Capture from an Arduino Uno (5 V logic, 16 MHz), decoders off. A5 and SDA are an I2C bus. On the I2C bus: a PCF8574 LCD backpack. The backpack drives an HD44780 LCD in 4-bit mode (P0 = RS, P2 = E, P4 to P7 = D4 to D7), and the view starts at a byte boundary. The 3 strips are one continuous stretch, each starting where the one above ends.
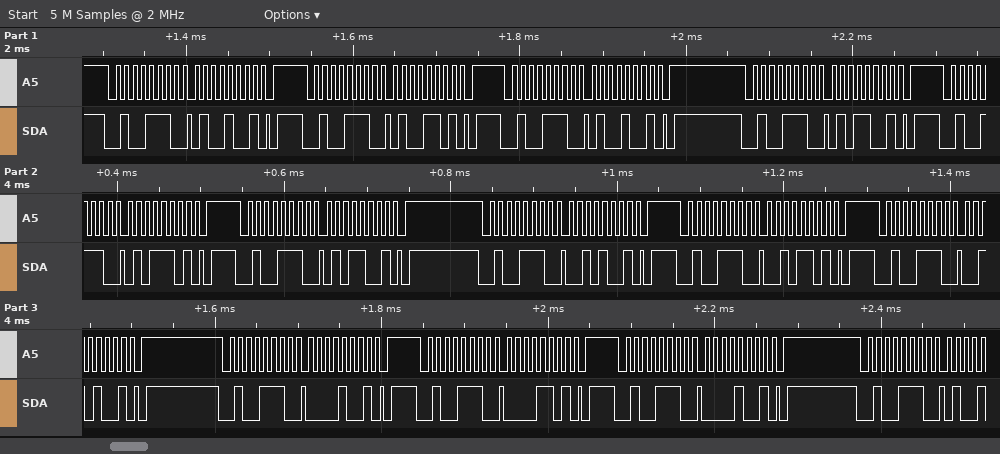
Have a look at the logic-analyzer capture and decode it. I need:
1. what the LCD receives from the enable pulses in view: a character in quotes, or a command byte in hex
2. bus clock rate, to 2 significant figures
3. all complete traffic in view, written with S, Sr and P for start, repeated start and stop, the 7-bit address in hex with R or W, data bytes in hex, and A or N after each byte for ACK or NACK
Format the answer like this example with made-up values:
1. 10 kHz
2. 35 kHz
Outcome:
1. 'E' ' '
2. 100 kHz
3. S 27W A 49 A P S 27W A 4D A P S 27W A 49 A P S 27W A 59 A P S 27W A 5D A P S 27W A 59 A P S 27W A 29 A P S 27W A 2D A P S 27W A 29 A P S 27W A 09 A P S 27W A 0D A P S 27W A 09 A P S 27W A
